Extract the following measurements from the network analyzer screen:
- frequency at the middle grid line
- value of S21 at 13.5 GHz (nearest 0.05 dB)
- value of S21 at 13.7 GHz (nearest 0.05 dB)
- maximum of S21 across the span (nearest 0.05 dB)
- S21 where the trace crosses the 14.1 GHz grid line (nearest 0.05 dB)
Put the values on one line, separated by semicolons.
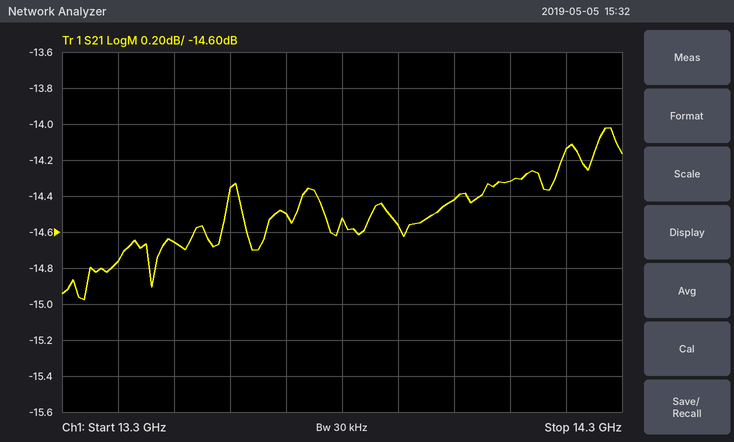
13.8 GHz; -14.65 dB; -14.50 dB; -14.00 dB; -14.30 dB
